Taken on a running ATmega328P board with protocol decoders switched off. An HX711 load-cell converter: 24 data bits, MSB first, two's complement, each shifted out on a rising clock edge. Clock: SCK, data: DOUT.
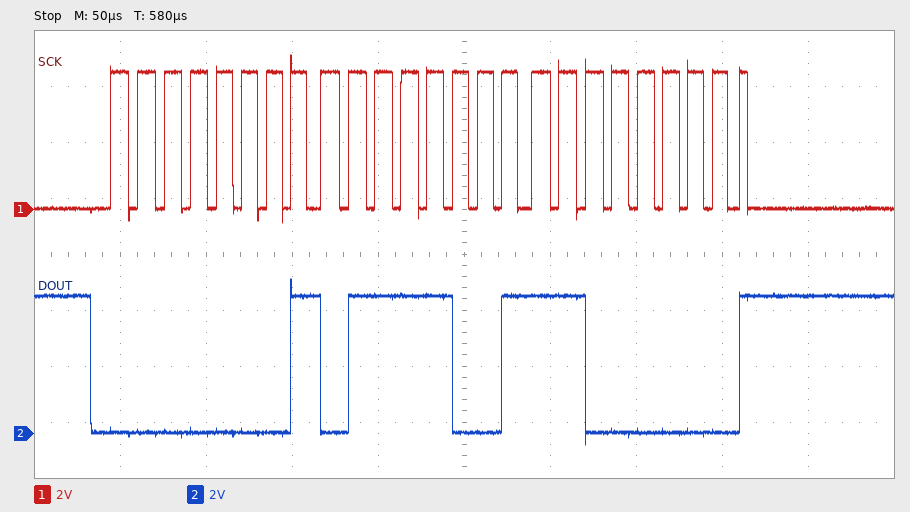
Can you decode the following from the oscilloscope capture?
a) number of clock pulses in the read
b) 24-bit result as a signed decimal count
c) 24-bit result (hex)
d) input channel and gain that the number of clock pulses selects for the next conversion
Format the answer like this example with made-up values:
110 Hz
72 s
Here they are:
25
96704
0x0179C0
channel A, gain 128
